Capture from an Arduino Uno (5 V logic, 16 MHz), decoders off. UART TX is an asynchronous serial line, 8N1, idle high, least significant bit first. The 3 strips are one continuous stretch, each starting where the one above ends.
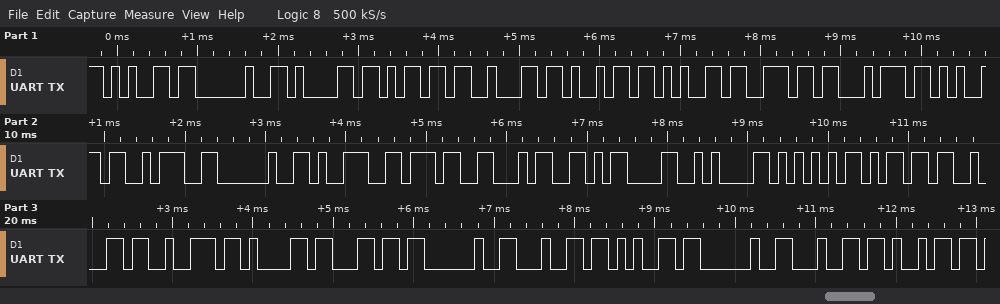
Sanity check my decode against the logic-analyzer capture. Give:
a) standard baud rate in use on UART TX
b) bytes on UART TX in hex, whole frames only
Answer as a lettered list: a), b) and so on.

a) 9600 baud
b) 65 20 61 6D 62 69 65 6E 74 65 3A 20 39 37 34 0D 0A 55 6D 62 72 61 6C 20 64 65 20 64 69
